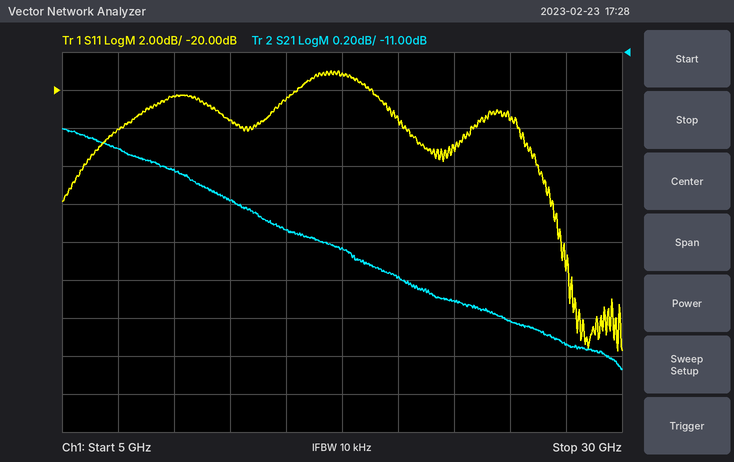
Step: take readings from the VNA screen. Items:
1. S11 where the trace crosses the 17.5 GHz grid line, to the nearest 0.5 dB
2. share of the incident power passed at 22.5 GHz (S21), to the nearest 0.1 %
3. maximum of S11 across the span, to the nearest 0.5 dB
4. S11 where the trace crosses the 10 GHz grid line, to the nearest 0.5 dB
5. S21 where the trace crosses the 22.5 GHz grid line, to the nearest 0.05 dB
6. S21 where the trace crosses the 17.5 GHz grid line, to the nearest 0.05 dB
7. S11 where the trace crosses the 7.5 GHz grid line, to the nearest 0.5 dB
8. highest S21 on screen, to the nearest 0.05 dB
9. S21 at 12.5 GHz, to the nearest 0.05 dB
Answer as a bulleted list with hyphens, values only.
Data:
- -19.0 dB
- 5.9 %
- -19.0 dB
- -20.5 dB
- -12.30 dB
- -12.05 dB
- -22.0 dB
- -11.40 dB
- -11.80 dB
